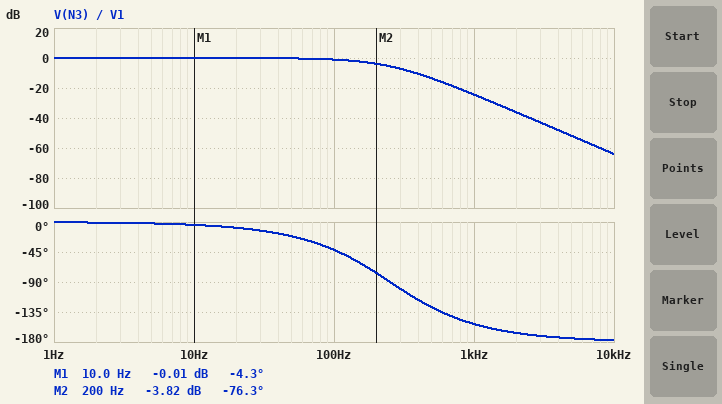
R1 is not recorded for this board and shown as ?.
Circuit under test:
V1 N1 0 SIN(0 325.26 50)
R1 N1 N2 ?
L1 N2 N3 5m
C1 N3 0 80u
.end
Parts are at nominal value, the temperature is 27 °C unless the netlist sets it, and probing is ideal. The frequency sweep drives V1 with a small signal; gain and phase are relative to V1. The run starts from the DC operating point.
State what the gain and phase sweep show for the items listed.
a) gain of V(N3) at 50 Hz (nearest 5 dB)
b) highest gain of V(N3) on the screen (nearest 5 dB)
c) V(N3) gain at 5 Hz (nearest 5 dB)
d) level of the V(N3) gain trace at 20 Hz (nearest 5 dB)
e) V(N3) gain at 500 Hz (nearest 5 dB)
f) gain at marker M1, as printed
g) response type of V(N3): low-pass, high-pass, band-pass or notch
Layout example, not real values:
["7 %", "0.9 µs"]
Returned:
["0 dB", "0 dB", "0 dB", "0 dB", "-15 dB", "-0.01 dB", "low-pass"]
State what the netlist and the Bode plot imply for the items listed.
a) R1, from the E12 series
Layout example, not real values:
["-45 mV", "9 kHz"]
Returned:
["15 Ω"]
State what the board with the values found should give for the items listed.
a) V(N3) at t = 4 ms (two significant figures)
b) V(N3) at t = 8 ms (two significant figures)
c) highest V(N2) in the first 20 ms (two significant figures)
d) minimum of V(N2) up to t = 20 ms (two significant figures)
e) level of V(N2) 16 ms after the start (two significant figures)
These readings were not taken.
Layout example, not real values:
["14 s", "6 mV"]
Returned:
["240 V", "270 V", "300 V", "-300 V", "-300 V"]
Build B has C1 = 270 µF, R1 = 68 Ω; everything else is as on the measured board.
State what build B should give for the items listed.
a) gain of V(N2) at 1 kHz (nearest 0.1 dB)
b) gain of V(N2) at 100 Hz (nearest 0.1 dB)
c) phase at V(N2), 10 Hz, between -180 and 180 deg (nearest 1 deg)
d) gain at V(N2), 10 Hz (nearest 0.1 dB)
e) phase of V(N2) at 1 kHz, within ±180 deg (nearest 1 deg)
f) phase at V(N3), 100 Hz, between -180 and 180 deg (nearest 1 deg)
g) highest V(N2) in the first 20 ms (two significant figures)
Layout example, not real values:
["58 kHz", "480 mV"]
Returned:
["-7.7 dB", "-27.9 dB", "-49 deg", "-3.7 dB", "66 deg", "-88 deg", "82 V"]
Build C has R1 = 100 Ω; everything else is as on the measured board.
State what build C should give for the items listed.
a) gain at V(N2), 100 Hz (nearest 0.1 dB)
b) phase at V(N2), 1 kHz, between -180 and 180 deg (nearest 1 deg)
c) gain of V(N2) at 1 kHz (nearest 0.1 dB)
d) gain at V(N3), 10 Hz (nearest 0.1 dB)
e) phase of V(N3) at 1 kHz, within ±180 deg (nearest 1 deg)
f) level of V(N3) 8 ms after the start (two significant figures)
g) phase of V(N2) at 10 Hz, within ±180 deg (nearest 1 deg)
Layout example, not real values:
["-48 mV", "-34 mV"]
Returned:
["-15.6 dB", "74 deg", "-11.0 dB", "-1.0 dB", "-106 deg", "160 V", "-27 deg"]
